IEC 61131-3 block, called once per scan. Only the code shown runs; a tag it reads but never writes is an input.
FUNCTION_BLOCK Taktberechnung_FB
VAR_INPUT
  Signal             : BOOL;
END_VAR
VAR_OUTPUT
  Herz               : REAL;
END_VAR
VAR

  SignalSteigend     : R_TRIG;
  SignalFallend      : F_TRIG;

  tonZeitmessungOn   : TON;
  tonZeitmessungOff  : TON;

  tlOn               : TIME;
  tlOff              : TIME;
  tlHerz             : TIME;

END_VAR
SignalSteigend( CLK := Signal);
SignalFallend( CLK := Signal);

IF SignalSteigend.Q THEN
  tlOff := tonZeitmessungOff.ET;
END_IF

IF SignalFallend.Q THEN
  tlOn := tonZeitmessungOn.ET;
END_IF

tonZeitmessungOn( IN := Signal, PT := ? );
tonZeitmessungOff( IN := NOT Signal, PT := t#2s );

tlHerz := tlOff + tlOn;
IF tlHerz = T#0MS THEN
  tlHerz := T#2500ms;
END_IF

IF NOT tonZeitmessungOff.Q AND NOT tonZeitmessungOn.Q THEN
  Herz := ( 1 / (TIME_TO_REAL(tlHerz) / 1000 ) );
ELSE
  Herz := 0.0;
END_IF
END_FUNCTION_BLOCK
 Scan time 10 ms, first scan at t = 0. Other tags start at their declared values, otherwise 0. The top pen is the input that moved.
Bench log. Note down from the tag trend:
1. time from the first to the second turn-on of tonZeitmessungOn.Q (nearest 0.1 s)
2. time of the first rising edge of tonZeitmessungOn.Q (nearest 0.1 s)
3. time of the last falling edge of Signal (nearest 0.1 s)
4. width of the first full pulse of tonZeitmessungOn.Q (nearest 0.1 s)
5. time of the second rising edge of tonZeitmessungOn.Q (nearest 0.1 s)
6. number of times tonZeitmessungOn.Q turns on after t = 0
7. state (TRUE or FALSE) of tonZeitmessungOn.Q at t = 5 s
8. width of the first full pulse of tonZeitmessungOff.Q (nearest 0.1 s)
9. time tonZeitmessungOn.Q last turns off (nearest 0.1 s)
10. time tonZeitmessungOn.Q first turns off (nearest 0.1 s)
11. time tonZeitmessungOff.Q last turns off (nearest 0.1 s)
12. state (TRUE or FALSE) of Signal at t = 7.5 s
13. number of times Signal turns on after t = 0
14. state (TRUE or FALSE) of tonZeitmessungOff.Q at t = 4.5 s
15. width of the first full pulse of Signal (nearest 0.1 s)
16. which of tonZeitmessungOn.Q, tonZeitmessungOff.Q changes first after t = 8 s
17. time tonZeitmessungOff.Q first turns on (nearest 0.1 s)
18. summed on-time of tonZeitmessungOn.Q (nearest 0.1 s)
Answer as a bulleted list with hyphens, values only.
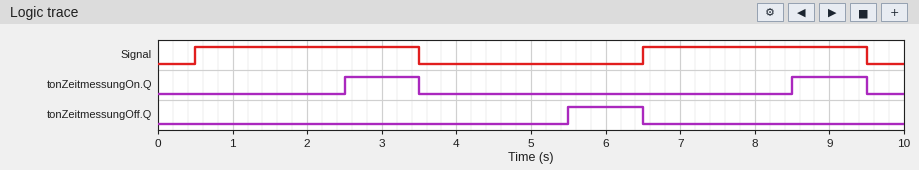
- 6.0 s
- 2.5 s
- 9.5 s
- 1.0 s
- 8.5 s
- 2
- FALSE
- 1.0 s
- 9.5 s
- 3.5 s
- 6.5 s
- TRUE
- 2
- FALSE
- 3.0 s
- tonZeitmessungOn.Q
- 5.5 s
- 2.0 s
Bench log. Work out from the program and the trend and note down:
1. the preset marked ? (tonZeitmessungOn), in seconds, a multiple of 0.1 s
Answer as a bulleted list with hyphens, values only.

- 2.0 s
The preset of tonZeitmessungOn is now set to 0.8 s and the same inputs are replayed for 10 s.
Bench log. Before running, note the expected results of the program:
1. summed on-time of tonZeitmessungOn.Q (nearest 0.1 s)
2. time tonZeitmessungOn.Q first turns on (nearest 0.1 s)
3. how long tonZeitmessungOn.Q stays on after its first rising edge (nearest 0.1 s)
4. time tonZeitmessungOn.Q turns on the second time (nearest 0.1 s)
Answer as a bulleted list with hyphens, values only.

- 4.4 s
- 1.3 s
- 2.2 s
- 7.3 s
